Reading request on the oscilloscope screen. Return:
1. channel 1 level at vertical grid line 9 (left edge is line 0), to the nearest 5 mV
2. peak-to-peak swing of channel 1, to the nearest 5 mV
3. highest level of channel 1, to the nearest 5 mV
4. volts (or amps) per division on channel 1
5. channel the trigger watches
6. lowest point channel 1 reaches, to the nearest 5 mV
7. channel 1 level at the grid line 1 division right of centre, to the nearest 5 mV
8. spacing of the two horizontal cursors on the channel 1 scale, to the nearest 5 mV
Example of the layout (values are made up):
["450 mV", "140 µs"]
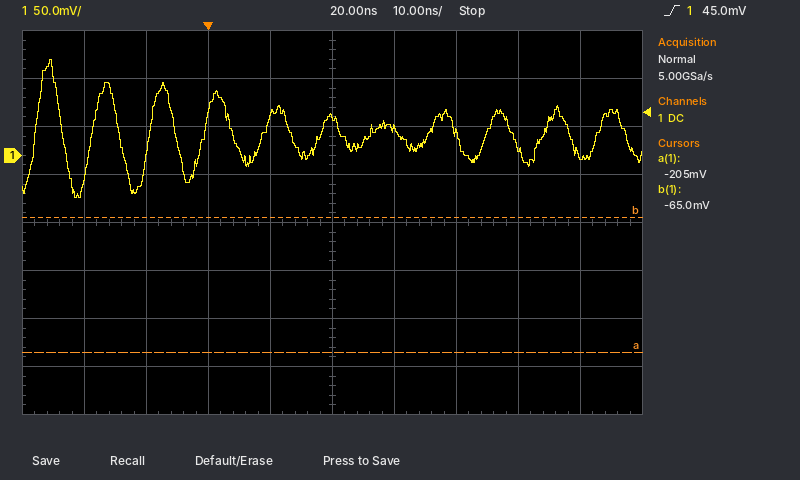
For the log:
["0 mV", "145 mV", "100 mV", "50 mV", "channel 1", "-45 mV", "30 mV", "140 mV"]
